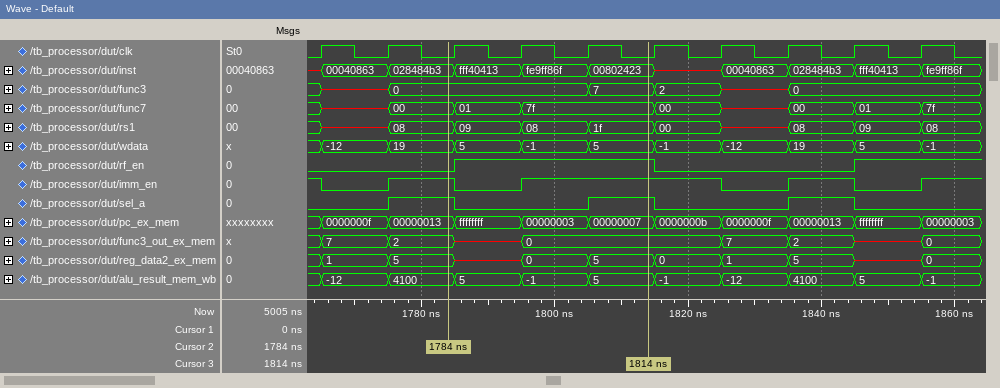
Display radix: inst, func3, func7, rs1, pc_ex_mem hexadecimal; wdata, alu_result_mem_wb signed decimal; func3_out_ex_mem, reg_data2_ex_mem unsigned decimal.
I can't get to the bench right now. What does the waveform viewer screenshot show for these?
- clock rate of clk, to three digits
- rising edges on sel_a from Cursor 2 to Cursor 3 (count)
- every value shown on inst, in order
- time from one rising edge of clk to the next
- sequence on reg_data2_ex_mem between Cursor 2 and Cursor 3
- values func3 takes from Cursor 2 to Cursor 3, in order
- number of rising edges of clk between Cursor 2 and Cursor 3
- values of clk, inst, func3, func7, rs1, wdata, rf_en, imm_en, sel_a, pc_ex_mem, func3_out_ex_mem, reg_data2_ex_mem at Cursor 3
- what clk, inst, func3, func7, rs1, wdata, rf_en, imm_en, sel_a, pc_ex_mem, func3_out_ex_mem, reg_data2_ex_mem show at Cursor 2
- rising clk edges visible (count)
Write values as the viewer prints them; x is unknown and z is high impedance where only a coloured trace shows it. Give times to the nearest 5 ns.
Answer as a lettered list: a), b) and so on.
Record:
a) 100 MHz
b) 1
c) x, 00040863, 028484b3, fff40413, fe9ff86f, 00802423, x, 00040863, 028484b3, fff40413, fe9ff86f
d) 10 ns
e) 5, x, 0, 5
f) 0, 7
g) 3
h) clk=0, inst=00802423, func3=7, func7=7f, rs1=1f, wdata=5, rf_en=1, imm_en=1, sel_a=1, pc_ex_mem=00000007, func3_out_ex_mem=0, reg_data2_ex_mem=5
i) clk=0, inst=028484b3, func3=0, func7=00, rs1=08, wdata=19, rf_en=0, imm_en=1, sel_a=1, pc_ex_mem=00000013, func3_out_ex_mem=2, reg_data2_ex_mem=5
j) 10
